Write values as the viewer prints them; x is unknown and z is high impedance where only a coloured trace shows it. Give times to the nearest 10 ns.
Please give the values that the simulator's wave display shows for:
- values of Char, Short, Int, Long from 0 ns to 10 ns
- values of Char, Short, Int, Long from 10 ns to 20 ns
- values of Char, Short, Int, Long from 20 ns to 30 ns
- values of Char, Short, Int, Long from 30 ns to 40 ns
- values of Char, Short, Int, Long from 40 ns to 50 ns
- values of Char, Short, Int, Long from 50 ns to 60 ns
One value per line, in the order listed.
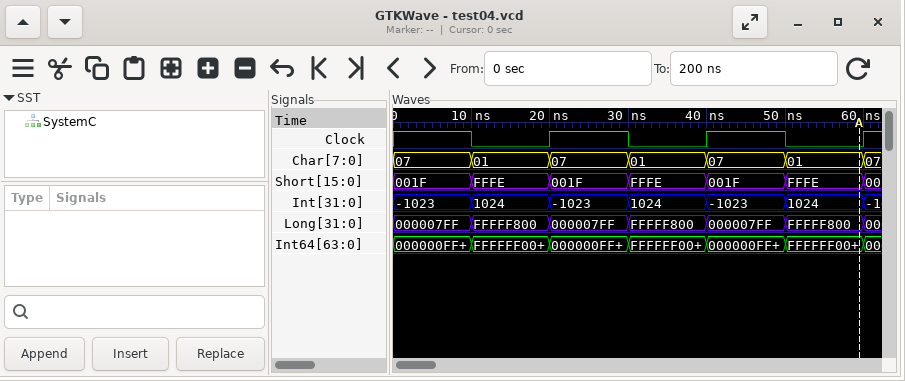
Char=07, Short=001F, Int=-1023, Long=000007FF
Char=01, Short=FFFE, Int=1024, Long=FFFFF800
Char=07, Short=001F, Int=-1023, Long=000007FF
Char=01, Short=FFFE, Int=1024, Long=FFFFF800
Char=07, Short=001F, Int=-1023, Long=000007FF
Char=01, Short=FFFE, Int=1024, Long=FFFFF800
